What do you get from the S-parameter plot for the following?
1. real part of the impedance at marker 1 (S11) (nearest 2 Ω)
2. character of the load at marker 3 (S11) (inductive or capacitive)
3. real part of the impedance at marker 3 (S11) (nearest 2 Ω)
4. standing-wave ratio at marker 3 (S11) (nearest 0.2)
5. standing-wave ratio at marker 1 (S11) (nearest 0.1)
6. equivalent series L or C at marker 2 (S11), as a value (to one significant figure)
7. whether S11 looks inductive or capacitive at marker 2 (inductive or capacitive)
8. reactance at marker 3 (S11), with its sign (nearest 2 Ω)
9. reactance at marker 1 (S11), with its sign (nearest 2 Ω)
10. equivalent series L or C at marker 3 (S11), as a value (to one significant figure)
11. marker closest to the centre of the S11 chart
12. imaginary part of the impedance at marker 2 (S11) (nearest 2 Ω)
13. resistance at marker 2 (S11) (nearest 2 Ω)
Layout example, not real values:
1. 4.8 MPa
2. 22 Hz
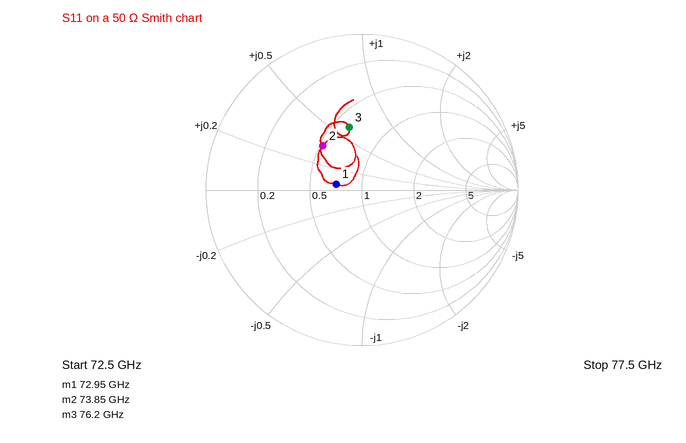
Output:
1. 36 Ω
2. inductive
3. 32 Ω
4. 2.4
5. 1.4
6. 40 pH
7. inductive
8. +30 Ω
9. +2 Ω
10. 60 pH
11. marker 1
12. +18 Ω
13. 26 Ω
